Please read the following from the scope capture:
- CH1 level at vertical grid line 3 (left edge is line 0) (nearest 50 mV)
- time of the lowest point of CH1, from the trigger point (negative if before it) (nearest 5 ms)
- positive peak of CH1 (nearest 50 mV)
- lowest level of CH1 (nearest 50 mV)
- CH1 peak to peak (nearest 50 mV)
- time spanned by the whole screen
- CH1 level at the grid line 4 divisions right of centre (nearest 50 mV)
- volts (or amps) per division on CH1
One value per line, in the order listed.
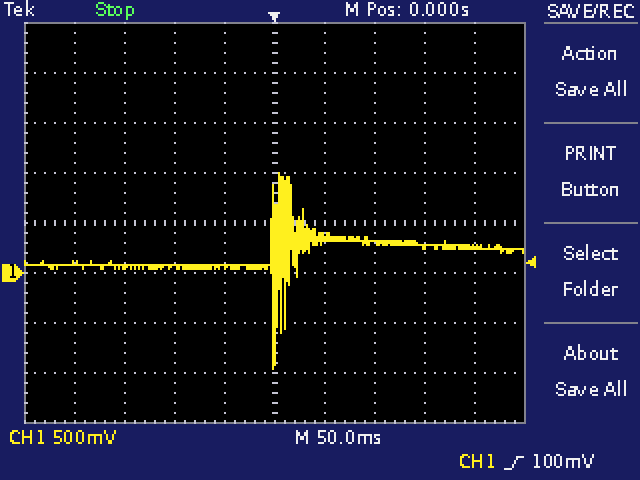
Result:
50 mV
0 ms
1.00 V
-950 mV
1.95 V
500 ms
250 mV
500 mV
